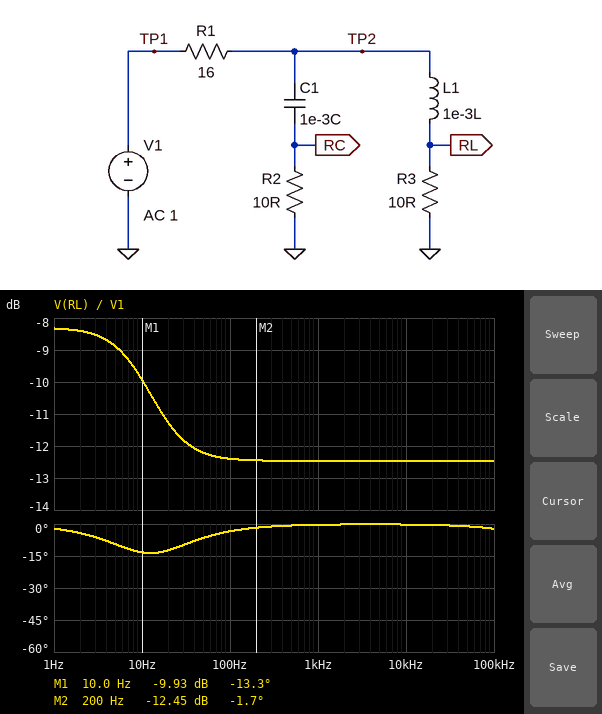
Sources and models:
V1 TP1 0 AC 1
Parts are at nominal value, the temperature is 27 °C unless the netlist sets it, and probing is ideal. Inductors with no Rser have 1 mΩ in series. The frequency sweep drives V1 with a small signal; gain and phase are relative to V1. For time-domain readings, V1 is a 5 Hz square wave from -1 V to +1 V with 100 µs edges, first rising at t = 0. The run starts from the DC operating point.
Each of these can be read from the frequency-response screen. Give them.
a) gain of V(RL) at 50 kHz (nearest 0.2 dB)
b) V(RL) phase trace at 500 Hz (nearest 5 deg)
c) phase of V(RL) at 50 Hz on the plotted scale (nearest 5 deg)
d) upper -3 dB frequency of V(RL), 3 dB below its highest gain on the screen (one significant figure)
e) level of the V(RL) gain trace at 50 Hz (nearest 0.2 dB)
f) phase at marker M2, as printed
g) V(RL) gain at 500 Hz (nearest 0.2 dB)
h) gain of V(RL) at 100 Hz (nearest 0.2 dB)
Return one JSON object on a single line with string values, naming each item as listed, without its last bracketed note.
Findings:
{"gain of V(RL) at 50 kHz": "-12.4 dB", "V(RL) phase trace at 500 Hz": "0 deg", "phase of V(RL) at 50 Hz on the plotted scale": "-5 deg", "upper -3 dB frequency of V(RL), 3 dB below its highest gain on the screen": "20 Hz", "level of the V(RL) gain trace at 50 Hz": "-12.2 dB", "phase at marker M2, as printed": "-1.7 deg", "V(RL) gain at 500 Hz": "-12.4 dB", "gain of V(RL) at 100 Hz": "-12.4 dB"}
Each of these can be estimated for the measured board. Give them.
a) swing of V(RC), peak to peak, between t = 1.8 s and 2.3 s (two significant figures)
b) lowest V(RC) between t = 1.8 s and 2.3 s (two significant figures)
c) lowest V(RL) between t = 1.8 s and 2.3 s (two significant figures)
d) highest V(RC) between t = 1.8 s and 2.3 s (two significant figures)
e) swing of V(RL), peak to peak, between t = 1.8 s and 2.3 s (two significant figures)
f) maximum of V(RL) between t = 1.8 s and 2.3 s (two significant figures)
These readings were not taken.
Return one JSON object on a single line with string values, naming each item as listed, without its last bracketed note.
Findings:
{"swing of V(RC), peak to peak, between t = 1.8 s and 2.3 s": "950 mV", "lowest V(RC) between t = 1.8 s and 2.3 s": "-470 mV", "lowest V(RL) between t = 1.8 s and 2.3 s": "-380 mV", "highest V(RC) between t = 1.8 s and 2.3 s": "470 mV", "swing of V(RL), peak to peak, between t = 1.8 s and 2.3 s": "770 mV", "maximum of V(RL) between t = 1.8 s and 2.3 s": "380 mV"}
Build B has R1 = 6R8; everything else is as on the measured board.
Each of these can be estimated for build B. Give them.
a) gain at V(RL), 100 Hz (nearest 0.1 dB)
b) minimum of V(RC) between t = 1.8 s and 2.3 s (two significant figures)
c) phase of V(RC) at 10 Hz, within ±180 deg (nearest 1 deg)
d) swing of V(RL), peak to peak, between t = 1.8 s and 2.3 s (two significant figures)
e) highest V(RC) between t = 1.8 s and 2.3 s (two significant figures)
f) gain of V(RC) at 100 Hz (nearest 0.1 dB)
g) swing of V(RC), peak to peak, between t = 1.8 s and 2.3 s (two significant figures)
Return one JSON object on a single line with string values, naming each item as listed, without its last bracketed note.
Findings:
{"gain at V(RL), 100 Hz": "-7.4 dB", "minimum of V(RC) between t = 1.8 s and 2.3 s": "-840 mV", "phase of V(RC) at 10 Hz, within ±180 deg": "49 deg", "swing of V(RL), peak to peak, between t = 1.8 s and 2.3 s": "1.2 V", "highest V(RC) between t = 1.8 s and 2.3 s": "840 mV", "gain of V(RC) at 100 Hz": "-7.5 dB", "swing of V(RC), peak to peak, between t = 1.8 s and 2.3 s": "1.7 V"}
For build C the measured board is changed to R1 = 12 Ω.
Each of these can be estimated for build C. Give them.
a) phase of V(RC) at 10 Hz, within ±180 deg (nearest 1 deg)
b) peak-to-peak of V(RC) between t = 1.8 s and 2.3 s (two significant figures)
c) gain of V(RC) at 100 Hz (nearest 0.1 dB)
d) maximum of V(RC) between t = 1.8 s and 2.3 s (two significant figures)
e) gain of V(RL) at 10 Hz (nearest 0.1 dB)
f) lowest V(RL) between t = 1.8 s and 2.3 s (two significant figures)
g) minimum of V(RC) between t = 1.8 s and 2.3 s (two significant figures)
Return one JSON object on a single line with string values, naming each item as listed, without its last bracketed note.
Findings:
{"phase of V(RC) at 10 Hz, within ±180 deg": "46 deg", "peak-to-peak of V(RC) between t = 1.8 s and 2.3 s": "1.2 V", "gain of V(RC) at 100 Hz": "-10.7 dB", "maximum of V(RC) between t = 1.8 s and 2.3 s": "590 mV", "gain of V(RL) at 10 Hz": "-8.3 dB", "lowest V(RL) between t = 1.8 s and 2.3 s": "-450 mV", "minimum of V(RC) between t = 1.8 s and 2.3 s": "-590 mV"}
